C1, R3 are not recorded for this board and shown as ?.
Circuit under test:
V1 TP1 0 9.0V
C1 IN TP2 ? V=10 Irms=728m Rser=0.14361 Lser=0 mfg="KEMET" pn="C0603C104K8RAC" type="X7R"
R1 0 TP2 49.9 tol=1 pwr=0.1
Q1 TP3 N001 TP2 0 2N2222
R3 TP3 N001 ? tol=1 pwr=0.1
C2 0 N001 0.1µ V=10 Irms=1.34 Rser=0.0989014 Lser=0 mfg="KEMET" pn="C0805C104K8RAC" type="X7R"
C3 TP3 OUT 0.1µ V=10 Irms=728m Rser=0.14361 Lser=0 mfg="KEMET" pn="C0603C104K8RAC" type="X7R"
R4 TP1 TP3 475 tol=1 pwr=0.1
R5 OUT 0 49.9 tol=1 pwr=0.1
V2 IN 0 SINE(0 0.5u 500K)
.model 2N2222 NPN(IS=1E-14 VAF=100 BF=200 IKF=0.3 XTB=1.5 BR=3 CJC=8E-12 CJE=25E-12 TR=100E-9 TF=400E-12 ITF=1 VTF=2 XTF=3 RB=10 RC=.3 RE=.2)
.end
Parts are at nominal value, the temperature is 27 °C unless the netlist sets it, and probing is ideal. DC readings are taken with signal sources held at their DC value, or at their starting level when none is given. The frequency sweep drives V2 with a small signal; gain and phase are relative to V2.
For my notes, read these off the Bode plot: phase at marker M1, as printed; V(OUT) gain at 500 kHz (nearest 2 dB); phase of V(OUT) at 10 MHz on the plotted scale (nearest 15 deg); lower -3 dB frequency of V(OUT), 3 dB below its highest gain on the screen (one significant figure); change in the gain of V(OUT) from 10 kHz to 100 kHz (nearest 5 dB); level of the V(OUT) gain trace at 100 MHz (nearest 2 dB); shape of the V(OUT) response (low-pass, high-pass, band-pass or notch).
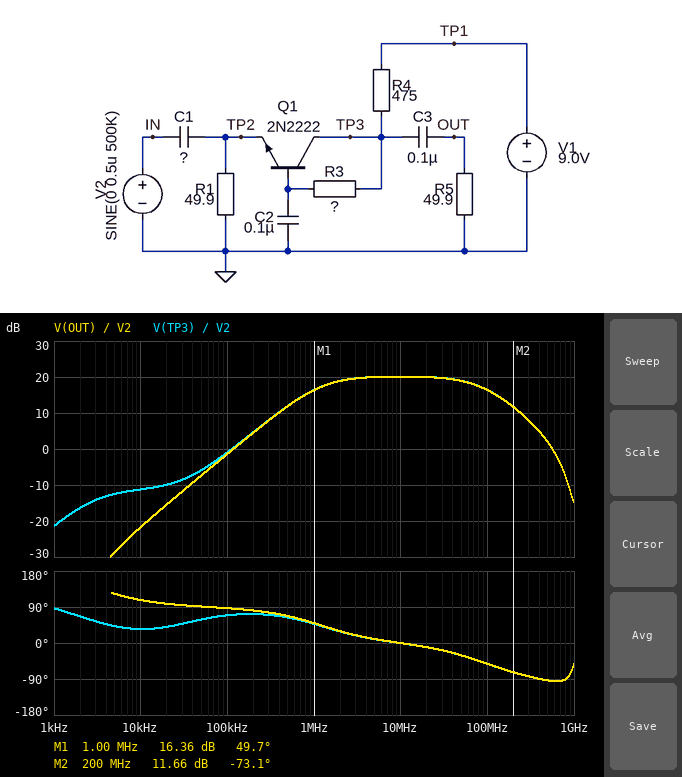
49.7 deg
12 dB
0 deg
1 MHz
20 dB
16 dB
band-pass
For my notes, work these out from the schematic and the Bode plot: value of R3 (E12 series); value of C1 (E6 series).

150 kΩ
33 nF
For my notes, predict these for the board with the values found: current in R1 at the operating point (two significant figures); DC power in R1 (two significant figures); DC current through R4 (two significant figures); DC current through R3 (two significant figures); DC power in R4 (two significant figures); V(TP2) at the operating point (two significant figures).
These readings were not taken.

6.6 mA
2.2 mW
6.6 mA
32 µA
21 mW
330 mV
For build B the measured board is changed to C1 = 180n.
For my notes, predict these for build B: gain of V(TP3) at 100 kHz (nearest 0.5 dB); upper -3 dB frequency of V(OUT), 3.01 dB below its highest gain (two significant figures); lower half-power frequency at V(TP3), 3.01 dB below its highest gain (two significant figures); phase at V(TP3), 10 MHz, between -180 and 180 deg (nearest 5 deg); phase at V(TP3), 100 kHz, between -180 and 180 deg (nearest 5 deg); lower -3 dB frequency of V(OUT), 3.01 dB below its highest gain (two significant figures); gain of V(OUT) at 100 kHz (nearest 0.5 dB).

13.0 dB
85 MHz
210 kHz
-5 deg
50 deg
220 kHz
12.5 dB
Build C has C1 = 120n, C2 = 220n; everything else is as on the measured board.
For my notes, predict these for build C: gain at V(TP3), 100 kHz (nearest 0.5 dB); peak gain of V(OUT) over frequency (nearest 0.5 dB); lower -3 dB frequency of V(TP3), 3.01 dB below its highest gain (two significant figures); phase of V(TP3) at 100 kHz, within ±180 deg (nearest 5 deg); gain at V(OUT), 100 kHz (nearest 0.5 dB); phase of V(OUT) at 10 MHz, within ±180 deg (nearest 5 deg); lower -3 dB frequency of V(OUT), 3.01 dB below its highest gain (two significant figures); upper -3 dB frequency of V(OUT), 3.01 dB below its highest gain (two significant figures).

10.0 dB
20.0 dB
320 kHz
55 deg
9.5 dB
-5 deg
330 kHz
85 MHz
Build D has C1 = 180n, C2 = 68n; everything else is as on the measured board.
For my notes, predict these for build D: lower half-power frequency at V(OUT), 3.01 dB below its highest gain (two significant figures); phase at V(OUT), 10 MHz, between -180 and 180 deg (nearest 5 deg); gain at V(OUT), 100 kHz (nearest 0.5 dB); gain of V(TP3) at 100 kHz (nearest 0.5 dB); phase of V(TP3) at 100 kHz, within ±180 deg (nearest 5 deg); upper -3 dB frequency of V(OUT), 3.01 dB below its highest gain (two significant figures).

220 kHz
-5 deg
12.5 dB
13.0 dB
50 deg
85 MHz
